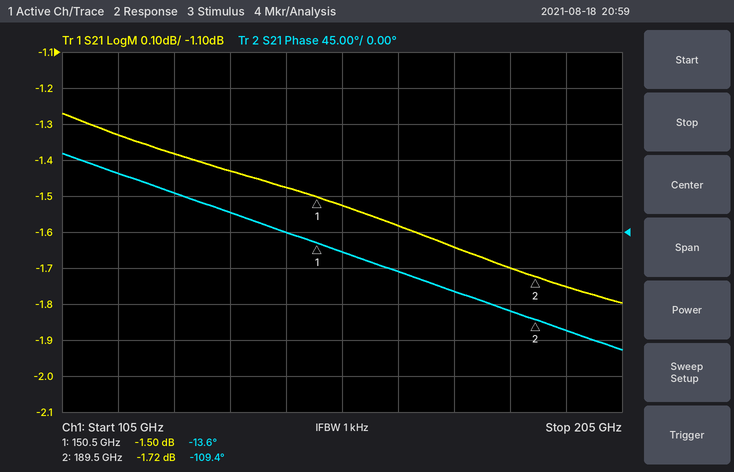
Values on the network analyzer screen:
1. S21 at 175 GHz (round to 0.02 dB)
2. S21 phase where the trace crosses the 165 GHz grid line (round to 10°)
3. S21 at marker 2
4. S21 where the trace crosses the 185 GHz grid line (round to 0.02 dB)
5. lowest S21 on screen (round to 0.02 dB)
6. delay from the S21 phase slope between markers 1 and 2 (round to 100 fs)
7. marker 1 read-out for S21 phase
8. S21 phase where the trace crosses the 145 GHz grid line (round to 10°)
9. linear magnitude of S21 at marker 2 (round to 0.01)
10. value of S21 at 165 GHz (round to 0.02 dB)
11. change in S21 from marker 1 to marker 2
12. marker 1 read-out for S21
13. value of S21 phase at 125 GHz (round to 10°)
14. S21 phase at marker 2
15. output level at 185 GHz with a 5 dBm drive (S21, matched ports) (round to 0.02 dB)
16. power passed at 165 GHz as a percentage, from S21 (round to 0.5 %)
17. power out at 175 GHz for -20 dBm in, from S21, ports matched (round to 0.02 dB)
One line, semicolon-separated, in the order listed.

-1.64 dB; -50°; -1.72 dB; -1.70 dB; -1.80 dB; 6.8 ps; -13.6°; 0°; 0.82; -1.58 dB; -0.22 dB; -1.50 dB; 50°; -109.4°; 3.30 dBm; 69.5 %; -21.64 dBm
